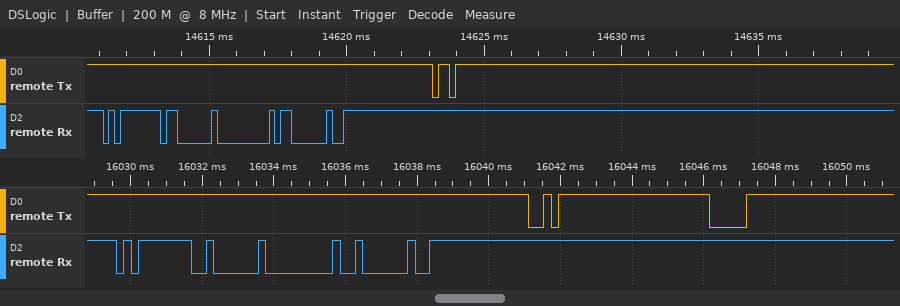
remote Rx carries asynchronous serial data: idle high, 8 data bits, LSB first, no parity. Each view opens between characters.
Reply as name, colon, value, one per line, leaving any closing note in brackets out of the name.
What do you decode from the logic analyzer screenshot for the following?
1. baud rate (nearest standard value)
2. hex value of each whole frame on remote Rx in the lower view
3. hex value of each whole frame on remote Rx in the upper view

baud rate: 4800 baud
hex value of each whole frame on remote Rx in the lower view: FD, 02, 00, 02, FE
hex value of each whole frame on remote Rx in the upper view: FD, 03, 00, 03, FE
